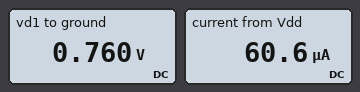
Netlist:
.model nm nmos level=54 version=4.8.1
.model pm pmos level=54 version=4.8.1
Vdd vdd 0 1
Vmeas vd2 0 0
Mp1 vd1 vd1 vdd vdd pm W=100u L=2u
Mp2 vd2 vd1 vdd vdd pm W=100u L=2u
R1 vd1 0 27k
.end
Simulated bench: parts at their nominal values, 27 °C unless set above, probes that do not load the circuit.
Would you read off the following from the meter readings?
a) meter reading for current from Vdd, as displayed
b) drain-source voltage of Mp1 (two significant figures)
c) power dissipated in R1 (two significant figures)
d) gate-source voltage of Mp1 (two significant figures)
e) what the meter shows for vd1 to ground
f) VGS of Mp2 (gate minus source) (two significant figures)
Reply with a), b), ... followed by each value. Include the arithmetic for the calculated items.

a) 60.6 µA
b) 760 mV - 1 V = -240 mV
c) (760 mV)^2 / 27 kΩ = 21 µW
d) 760 mV - 1 V = -240 mV
e) 0.760 V
f) 760 mV - 1 V = -240 mV
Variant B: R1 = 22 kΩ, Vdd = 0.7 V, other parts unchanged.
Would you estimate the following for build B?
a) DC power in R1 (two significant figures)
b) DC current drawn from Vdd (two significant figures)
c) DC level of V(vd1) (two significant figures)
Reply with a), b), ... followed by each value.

a) 10 µW
b) 45 µA
c) 470 mV
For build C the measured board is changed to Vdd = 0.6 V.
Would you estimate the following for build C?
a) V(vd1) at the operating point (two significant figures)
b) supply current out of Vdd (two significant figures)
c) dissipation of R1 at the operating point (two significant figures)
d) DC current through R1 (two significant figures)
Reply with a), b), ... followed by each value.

a) 390 mV
b) 30 µA
c) 5.6 µW
d) 14 µA
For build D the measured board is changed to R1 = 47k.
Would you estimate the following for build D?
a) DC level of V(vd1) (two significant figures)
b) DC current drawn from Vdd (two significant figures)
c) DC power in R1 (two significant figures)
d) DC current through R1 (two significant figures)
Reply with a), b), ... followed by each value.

a) 780 mV
b) 36 µA
c) 13 µW
d) 17 µA
